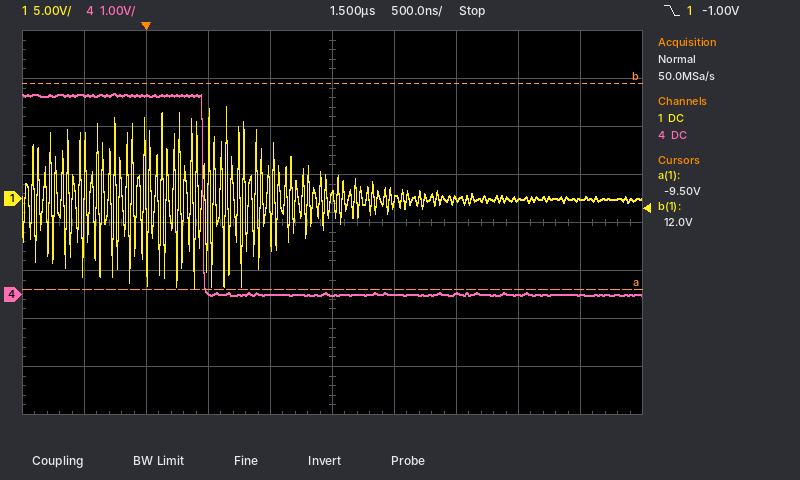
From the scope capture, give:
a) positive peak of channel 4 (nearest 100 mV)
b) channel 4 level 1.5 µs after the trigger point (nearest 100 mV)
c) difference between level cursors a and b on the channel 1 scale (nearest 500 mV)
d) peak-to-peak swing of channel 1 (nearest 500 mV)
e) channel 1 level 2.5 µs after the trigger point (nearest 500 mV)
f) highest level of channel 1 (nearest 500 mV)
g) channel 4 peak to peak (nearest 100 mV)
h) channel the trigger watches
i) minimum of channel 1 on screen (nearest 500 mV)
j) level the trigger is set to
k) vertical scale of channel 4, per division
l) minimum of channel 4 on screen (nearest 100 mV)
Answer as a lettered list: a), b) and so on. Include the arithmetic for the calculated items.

a) 4.2 V
b) 0.0 V
c) 21.5 V
d) 9.5 V − (-9.5 V) = 19.0 V
e) 0.0 V
f) 9.5 V
g) 4.2 V − (0.0 V) = 4.2 V
h) channel 1
i) -9.5 V
j) -1.00 V
k) 1 V
l) 0.0 V
